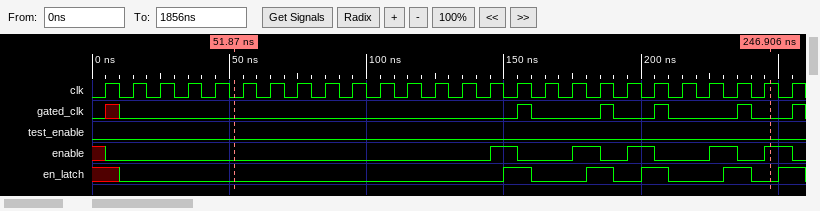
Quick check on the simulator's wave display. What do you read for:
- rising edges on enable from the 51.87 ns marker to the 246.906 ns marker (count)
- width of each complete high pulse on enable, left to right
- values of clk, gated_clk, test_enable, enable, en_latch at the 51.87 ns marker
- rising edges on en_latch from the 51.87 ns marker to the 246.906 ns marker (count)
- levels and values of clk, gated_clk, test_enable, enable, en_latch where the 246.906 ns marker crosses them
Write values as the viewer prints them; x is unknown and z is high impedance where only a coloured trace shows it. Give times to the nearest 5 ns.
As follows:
5
10 ns, 10 ns, 10 ns, 10 ns, 10 ns
clk=0, gated_clk=0, test_enable=0, enable=0, en_latch=0
4
clk=1, gated_clk=0, test_enable=0, enable=1, en_latch=0
